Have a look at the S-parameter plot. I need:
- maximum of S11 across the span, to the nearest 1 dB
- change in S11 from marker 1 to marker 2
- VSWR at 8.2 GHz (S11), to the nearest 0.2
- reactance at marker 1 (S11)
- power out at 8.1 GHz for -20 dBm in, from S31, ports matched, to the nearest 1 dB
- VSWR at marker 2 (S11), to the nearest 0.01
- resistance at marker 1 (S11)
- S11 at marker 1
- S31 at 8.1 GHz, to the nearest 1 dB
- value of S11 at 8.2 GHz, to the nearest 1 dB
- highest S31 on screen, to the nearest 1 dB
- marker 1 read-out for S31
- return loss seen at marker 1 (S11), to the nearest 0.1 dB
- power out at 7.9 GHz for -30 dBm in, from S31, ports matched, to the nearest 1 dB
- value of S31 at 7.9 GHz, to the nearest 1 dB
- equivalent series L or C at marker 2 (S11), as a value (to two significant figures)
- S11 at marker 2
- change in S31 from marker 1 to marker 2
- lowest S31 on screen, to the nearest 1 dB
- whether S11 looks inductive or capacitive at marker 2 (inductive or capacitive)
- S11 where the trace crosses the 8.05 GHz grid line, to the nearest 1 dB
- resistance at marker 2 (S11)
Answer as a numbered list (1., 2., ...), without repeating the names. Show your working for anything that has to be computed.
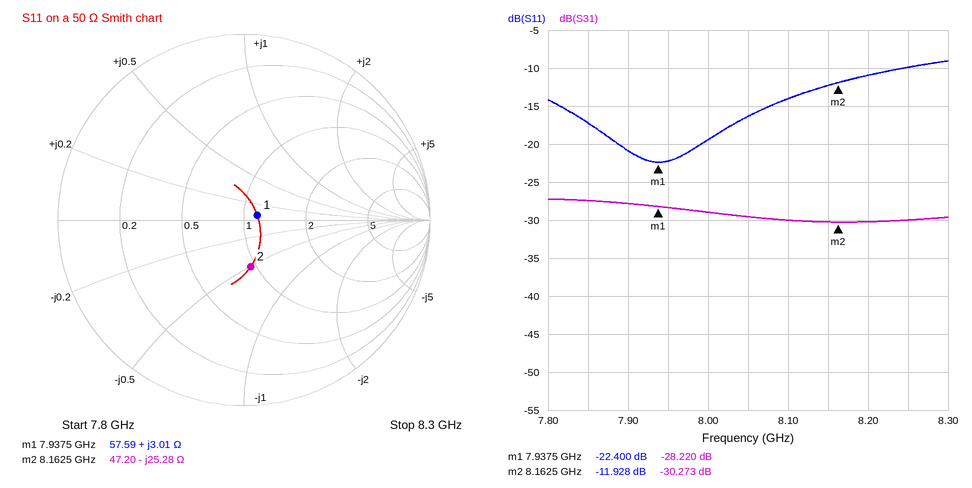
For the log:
1. -9 dB
2. -11.928 − (-22.4) = 10.472 dB
3. |Γ| = 10^(-11/20) = 0.2818; VSWR = (1 + 0.2818)/(1 − 0.2818) ≈ 1.8
4. +3.01 Ω
5. -20 dBm + (-30 dB) = -50 dBm
6. 1.68
7. 57.59 Ω
8. -22.400 dB
9. -30 dB
10. -11 dB
11. -27 dB
12. -28.220 dB
13. 22.4 dB
14. -30 dBm + (-28 dB) = -58 dBm
15. -28 dB
16. C = 1/(2π × 8.1625 GHz × 25.28 Ω) ≈ 771 fF, so 770 fF to two significant figures
17. -11.928 dB
18. -30.273 − (-28.22) = -2.053 dB
19. -30 dB
20. capacitive
21. -16 dB
22. 47.20 Ω
